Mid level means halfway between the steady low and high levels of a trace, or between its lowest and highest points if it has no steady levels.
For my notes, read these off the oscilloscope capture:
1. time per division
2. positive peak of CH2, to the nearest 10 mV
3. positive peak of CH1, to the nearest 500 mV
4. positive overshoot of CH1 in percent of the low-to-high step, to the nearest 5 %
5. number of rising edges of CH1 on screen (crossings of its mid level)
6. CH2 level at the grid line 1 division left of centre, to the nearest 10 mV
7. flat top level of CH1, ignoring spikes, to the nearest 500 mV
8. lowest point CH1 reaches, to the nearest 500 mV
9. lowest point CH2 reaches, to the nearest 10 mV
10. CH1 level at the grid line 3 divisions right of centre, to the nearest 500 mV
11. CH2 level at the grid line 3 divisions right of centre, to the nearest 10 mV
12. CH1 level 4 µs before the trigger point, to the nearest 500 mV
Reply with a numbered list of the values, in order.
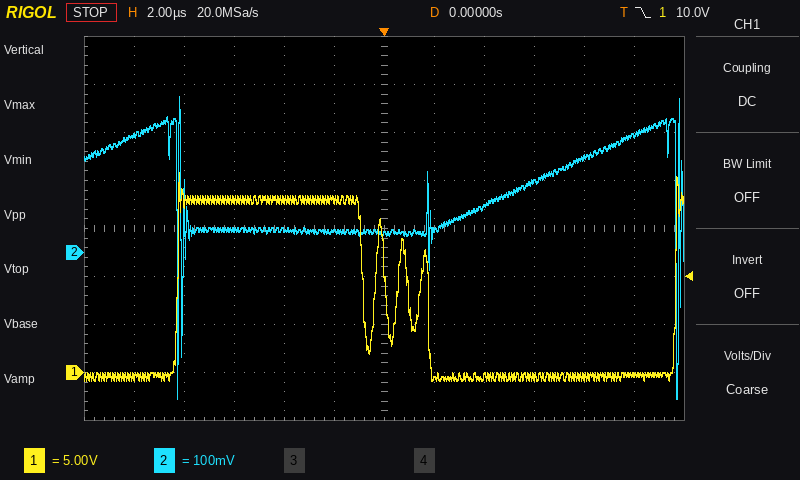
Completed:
1. 2 µs
2. 320 mV
3. 21.0 V
4. 15 %
5. 5
6. 40 mV
7. 18.0 V
8. -1.0 V
9. -300 mV
10. -500 mV
11. 150 mV
12. 18.0 V
